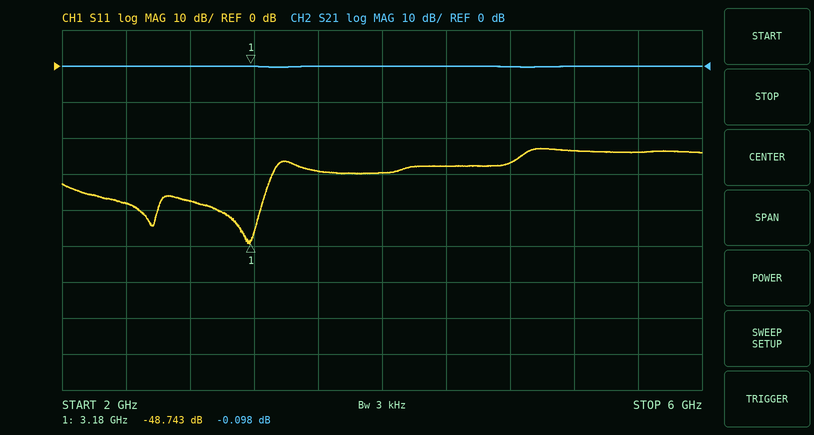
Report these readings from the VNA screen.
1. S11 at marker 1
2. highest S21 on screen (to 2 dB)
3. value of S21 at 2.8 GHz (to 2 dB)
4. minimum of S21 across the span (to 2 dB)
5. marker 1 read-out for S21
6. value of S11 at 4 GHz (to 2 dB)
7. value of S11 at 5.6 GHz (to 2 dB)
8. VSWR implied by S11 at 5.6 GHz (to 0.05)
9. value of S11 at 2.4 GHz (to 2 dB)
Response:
-48.743 dB
0 dB
0 dB
0 dB
-0.098 dB
-30 dB
-24 dB
1.15
-38 dB
